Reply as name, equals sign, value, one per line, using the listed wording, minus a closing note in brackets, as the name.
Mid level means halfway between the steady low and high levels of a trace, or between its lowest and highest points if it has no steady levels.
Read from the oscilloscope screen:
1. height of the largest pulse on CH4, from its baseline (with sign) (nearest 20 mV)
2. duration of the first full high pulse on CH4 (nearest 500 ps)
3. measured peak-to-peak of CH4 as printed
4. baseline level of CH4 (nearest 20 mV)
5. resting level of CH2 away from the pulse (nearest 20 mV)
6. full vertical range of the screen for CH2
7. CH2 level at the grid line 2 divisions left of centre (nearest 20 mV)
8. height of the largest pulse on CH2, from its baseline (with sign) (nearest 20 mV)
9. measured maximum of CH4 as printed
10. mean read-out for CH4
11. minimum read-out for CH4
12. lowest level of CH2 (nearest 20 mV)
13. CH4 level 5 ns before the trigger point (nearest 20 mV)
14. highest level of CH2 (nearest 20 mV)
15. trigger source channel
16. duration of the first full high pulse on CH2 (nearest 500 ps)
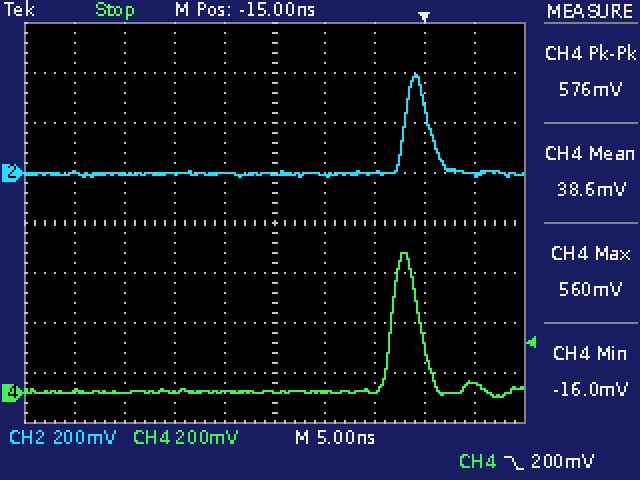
height of the largest pulse on CH4, from its baseline (with sign) = +560 mV
duration of the first full high pulse on CH4 = 3.0 ns
measured peak-to-peak of CH4 as printed = 576 mV
baseline level of CH4 = 0 mV
resting level of CH2 away from the pulse = 0 mV
full vertical range of the screen for CH2 = 1.6 V
CH2 level at the grid line 2 divisions left of centre = 0 mV
height of the largest pulse on CH2, from its baseline (with sign) = +400 mV
measured maximum of CH4 as printed = 560 mV
mean read-out for CH4 = 38.6 mV
minimum read-out for CH4 = -16.0 mV
lowest level of CH2 = -20 mV
CH4 level 5 ns before the trigger point = 0 mV
highest level of CH2 = 400 mV
trigger source channel = CH4
duration of the first full high pulse on CH2 = 2.5 ns
